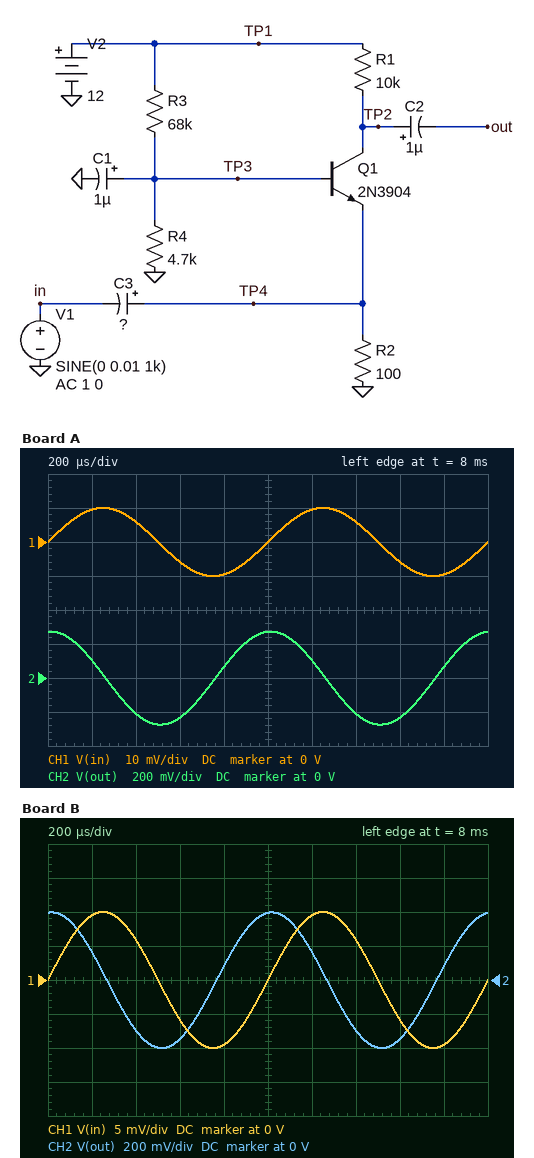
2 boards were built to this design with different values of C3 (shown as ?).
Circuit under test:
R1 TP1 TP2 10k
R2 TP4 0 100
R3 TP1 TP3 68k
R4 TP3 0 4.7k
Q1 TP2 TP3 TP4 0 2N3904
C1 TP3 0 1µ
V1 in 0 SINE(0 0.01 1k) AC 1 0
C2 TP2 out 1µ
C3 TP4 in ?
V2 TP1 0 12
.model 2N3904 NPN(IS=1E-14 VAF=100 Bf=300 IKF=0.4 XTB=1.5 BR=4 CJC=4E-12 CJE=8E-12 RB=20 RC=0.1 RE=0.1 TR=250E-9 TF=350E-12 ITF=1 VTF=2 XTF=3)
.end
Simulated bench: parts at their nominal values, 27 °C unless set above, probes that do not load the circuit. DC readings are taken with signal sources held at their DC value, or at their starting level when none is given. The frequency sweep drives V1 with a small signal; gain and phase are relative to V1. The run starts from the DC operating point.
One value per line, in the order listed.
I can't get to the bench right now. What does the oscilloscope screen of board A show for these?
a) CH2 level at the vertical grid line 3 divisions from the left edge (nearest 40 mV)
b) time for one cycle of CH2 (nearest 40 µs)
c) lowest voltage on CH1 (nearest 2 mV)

-240 mV
1.00 ms
-10 mV
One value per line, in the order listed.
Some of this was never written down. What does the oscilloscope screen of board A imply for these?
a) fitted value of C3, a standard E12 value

560 nF
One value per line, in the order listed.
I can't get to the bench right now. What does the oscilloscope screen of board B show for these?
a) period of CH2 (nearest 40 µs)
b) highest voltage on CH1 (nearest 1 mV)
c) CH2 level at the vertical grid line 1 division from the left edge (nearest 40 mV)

1.00 ms
10 mV
160 mV
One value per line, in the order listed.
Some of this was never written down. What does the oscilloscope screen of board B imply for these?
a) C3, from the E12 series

820 nF
